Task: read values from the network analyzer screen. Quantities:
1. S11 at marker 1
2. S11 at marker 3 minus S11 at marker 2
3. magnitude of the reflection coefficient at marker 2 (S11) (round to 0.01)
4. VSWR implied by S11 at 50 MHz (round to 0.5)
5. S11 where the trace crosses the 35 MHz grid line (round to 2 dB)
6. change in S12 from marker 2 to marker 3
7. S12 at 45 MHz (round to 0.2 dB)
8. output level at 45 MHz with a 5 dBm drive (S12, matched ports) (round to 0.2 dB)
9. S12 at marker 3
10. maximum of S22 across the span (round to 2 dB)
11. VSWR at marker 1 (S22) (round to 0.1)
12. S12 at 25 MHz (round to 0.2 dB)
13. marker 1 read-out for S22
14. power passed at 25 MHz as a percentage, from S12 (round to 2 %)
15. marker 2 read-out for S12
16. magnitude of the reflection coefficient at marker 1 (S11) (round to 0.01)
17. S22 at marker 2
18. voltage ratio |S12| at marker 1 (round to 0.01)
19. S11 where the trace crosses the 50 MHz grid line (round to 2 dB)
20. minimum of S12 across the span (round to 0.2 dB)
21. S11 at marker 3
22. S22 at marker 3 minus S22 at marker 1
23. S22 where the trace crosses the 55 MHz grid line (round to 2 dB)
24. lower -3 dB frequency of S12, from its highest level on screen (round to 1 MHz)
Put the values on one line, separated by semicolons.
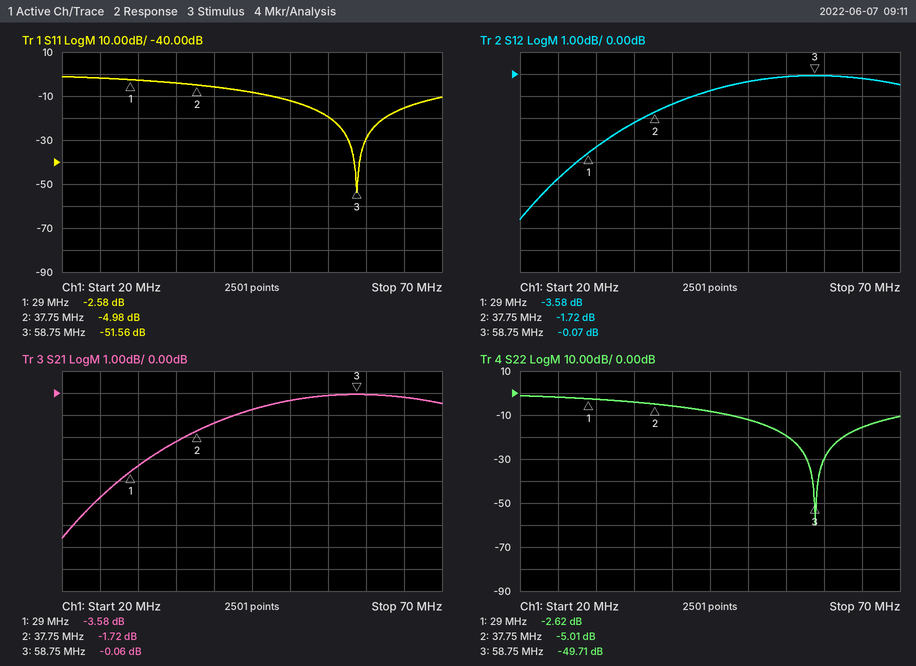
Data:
-2.58 dB; -46.58 dB; 0.56; 1.5; -4 dB; 1.65 dB; -0.8 dB; 4.2 dBm; -0.07 dB; -2 dB; 6.7; -4.8 dB; -2.62 dB; 34 %; -1.72 dB; 0.74; -5.01 dB; 0.66; -12 dB; -6.6 dB; -51.56 dB; -47.09 dB; -20 dB; 31 MHz
